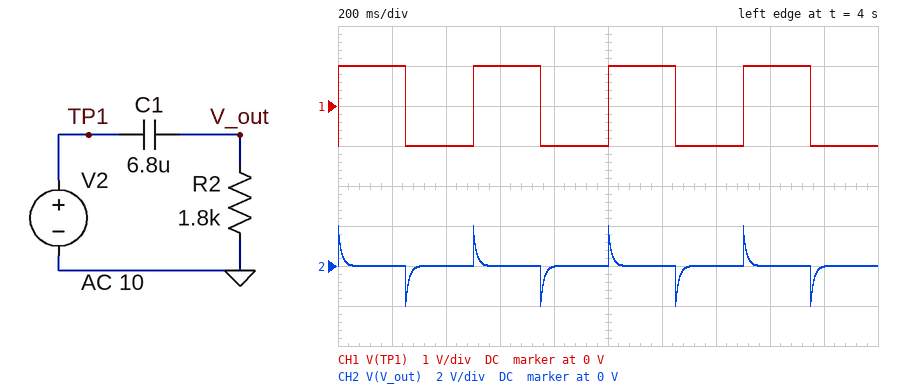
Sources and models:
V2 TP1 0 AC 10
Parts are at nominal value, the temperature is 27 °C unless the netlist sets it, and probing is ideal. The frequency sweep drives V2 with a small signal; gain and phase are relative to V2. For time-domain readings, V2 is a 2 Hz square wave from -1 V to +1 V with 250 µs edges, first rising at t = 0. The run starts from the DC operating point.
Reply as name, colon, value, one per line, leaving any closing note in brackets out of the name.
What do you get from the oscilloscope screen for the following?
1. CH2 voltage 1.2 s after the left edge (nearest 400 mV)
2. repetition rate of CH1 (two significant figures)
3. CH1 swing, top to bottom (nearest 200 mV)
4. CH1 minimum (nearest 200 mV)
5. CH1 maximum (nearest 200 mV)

CH2 voltage 1.2 s after the left edge: 0 V
repetition rate of CH1: 2.0 Hz
CH1 swing, top to bottom: 2.0 V
CH1 minimum: -1.0 V
CH1 maximum: 1.0 V
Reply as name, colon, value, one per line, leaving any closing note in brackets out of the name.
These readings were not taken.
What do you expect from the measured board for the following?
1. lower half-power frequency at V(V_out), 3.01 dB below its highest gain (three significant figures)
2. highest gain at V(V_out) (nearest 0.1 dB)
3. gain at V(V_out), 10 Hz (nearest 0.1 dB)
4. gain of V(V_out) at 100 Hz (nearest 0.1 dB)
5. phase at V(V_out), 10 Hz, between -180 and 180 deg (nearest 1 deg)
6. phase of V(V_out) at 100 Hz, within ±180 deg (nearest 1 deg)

lower half-power frequency at V(V_out), 3.01 dB below its highest gain: 13.0 Hz
highest gain at V(V_out): 0 dB
gain at V(V_out), 10 Hz: -4.3 dB
gain of V(V_out) at 100 Hz: -0.1 dB
phase at V(V_out), 10 Hz, between -180 and 180 deg: 52 deg
phase of V(V_out) at 100 Hz, within ±180 deg: 7 deg
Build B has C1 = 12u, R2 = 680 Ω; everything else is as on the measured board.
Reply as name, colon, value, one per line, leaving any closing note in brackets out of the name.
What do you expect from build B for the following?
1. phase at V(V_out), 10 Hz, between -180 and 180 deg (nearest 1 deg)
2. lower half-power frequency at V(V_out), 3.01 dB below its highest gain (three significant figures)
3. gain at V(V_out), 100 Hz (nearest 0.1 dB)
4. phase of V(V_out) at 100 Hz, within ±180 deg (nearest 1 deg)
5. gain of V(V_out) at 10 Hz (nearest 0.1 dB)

phase at V(V_out), 10 Hz, between -180 and 180 deg: 63 deg
lower half-power frequency at V(V_out), 3.01 dB below its highest gain: 19.5 Hz
gain at V(V_out), 100 Hz: -0.2 dB
phase of V(V_out) at 100 Hz, within ±180 deg: 11 deg
gain of V(V_out) at 10 Hz: -6.8 dB
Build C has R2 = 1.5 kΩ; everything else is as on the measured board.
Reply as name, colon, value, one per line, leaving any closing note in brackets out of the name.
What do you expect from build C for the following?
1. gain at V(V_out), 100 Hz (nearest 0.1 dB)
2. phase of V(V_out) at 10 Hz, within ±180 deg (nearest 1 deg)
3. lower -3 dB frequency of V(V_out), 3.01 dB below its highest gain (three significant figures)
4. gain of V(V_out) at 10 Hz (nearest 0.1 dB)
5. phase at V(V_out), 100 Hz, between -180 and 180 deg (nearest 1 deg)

gain at V(V_out), 100 Hz: -0.1 dB
phase of V(V_out) at 10 Hz, within ±180 deg: 57 deg
lower -3 dB frequency of V(V_out), 3.01 dB below its highest gain: 15.6 Hz
gain of V(V_out) at 10 Hz: -5.4 dB
phase at V(V_out), 100 Hz, between -180 and 180 deg: 9 deg
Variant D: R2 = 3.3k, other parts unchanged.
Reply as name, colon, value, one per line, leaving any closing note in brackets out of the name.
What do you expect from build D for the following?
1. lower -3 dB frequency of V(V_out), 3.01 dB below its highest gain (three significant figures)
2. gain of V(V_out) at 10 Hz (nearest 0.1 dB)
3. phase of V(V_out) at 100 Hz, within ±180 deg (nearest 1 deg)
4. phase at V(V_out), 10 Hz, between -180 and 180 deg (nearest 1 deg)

lower -3 dB frequency of V(V_out), 3.01 dB below its highest gain: 7.09 Hz
gain of V(V_out) at 10 Hz: -1.8 dB
phase of V(V_out) at 100 Hz, within ±180 deg: 4 deg
phase at V(V_out), 10 Hz, between -180 and 180 deg: 35 deg
